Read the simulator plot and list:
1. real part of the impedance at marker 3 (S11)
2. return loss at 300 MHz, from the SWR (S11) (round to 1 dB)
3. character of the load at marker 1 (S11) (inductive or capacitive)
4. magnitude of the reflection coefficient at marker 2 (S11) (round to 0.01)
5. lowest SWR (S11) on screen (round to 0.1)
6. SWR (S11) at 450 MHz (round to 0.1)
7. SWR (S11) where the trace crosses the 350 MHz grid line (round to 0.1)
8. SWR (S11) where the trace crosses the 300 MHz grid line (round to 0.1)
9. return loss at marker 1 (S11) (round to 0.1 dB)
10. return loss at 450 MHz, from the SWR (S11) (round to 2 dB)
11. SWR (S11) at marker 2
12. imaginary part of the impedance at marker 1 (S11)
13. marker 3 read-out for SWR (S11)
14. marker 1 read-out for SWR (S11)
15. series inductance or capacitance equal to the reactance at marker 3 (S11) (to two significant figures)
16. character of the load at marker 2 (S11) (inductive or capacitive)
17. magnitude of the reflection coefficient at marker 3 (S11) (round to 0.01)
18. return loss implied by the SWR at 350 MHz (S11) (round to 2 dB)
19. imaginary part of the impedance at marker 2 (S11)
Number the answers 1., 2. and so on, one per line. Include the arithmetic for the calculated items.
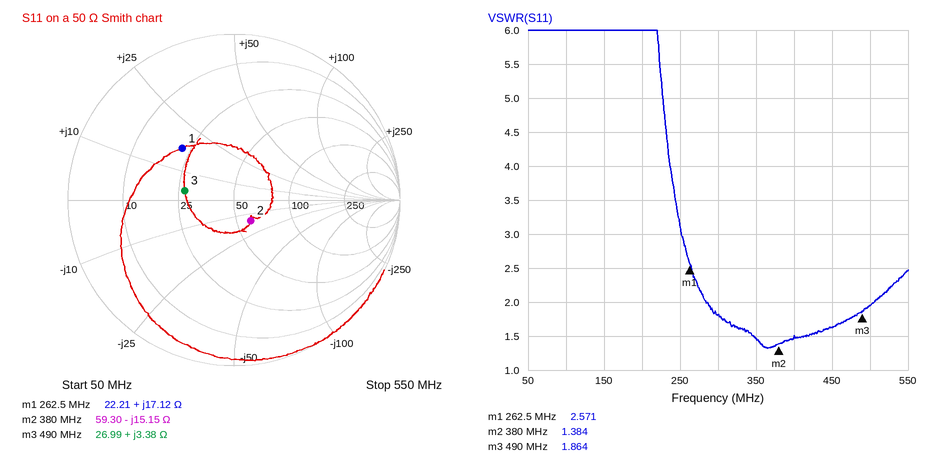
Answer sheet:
1. 26.99 Ω
2. −20 log10((1.8 − 1)/(1.8 + 1)) ≈ 11 dB
3. inductive
4. 0.16
5. 1.3
6. 1.6
7. 1.5
8. 1.8
9. 7.1 dB
10. −20 log10((1.6 − 1)/(1.6 + 1)) ≈ 12.7 dB, so 12 dB to the nearest 2 dB
11. 1.384
12. +17.12 Ω
13. 1.864
14. 2.571
15. L = 3.38 Ω/(2π × 490 MHz) ≈ 1.1 nH
16. capacitive
17. 0.30
18. −20 log10((1.5 − 1)/(1.5 + 1)) ≈ 14 dB
19. -15.15 Ω
